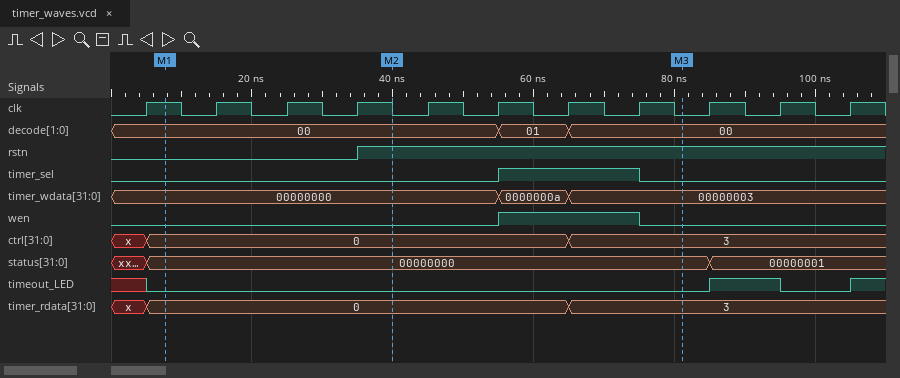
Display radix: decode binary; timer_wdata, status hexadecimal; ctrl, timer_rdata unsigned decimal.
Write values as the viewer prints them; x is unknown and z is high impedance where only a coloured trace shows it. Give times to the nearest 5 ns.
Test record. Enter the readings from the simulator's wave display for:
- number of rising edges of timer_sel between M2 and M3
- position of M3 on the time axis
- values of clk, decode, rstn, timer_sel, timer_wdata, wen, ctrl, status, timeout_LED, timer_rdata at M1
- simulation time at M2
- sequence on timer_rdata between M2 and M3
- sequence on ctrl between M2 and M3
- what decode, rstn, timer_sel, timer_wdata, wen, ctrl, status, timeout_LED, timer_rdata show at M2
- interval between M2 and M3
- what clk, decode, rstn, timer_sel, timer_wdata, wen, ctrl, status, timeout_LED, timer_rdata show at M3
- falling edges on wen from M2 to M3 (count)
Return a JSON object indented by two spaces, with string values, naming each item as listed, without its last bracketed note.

{
  "number of rising edges of timer_sel between M2 and M3": "1",
  "position of M3 on the time axis": "80 ns",
  "values of clk, decode, rstn, timer_sel, timer_wdata, wen, ctrl, status, timeout_LED, timer_rdata at M1": "clk=1, decode=00, rstn=0, timer_sel=0, timer_wdata=00000000, wen=0, ctrl=0, status=00000000, timeout_LED=0, timer_rdata=0",
  "simulation time at M2": "40 ns",
  "sequence on timer_rdata between M2 and M3": "0, 3",
  "sequence on ctrl between M2 and M3": "0, 3",
  "what decode, rstn, timer_sel, timer_wdata, wen, ctrl, status, timeout_LED, timer_rdata show at M2": "decode=00, rstn=1, timer_sel=0, timer_wdata=00000000, wen=0, ctrl=0, status=00000000, timeout_LED=0, timer_rdata=0",
  "interval between M2 and M3": "40 ns",
  "what clk, decode, rstn, timer_sel, timer_wdata, wen, ctrl, status, timeout_LED, timer_rdata show at M3": "clk=0, decode=00, rstn=1, timer_sel=0, timer_wdata=00000003, wen=0, ctrl=3, status=00000000, timeout_LED=0, timer_rdata=3",
  "falling edges on wen from M2 to M3": "1"
}
